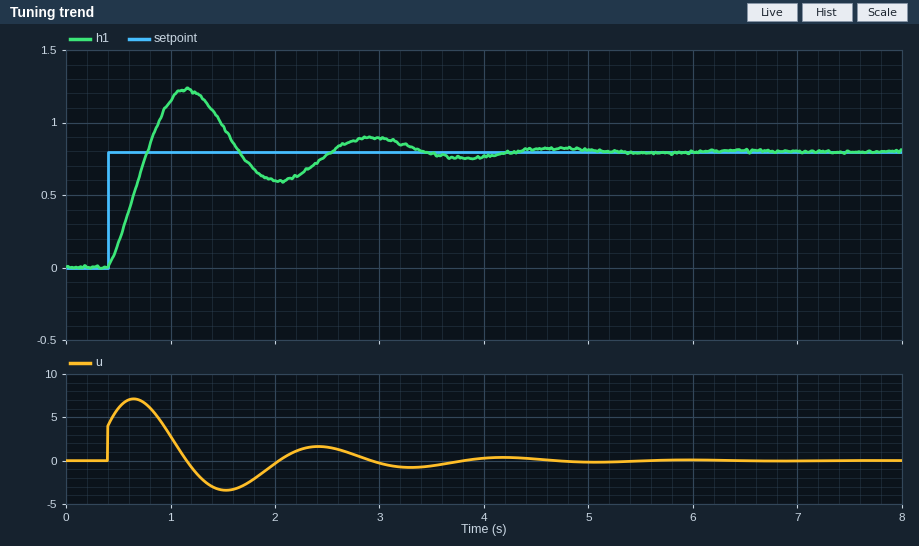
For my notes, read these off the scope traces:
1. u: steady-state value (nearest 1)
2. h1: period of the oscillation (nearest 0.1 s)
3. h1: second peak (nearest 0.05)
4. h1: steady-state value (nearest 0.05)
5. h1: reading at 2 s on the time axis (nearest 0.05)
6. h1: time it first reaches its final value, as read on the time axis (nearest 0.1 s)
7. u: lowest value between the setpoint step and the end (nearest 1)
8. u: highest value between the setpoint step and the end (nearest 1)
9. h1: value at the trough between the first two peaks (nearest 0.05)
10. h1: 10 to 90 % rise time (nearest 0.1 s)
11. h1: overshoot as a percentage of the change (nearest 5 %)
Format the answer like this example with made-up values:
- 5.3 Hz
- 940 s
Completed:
- 0
- 1.8 s
- 0.90
- 0.80
- 0.60
- 0.8 s
- -3
- 7
- 0.60
- 0.3 s
- 55 %
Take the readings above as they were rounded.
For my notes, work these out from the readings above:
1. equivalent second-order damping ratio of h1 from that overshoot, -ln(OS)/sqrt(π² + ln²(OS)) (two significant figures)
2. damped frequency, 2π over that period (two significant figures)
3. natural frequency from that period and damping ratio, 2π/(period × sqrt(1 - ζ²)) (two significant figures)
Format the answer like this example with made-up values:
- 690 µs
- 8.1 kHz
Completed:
- 0.19
- 3.5 rad/s
- 3.6 rad/s
